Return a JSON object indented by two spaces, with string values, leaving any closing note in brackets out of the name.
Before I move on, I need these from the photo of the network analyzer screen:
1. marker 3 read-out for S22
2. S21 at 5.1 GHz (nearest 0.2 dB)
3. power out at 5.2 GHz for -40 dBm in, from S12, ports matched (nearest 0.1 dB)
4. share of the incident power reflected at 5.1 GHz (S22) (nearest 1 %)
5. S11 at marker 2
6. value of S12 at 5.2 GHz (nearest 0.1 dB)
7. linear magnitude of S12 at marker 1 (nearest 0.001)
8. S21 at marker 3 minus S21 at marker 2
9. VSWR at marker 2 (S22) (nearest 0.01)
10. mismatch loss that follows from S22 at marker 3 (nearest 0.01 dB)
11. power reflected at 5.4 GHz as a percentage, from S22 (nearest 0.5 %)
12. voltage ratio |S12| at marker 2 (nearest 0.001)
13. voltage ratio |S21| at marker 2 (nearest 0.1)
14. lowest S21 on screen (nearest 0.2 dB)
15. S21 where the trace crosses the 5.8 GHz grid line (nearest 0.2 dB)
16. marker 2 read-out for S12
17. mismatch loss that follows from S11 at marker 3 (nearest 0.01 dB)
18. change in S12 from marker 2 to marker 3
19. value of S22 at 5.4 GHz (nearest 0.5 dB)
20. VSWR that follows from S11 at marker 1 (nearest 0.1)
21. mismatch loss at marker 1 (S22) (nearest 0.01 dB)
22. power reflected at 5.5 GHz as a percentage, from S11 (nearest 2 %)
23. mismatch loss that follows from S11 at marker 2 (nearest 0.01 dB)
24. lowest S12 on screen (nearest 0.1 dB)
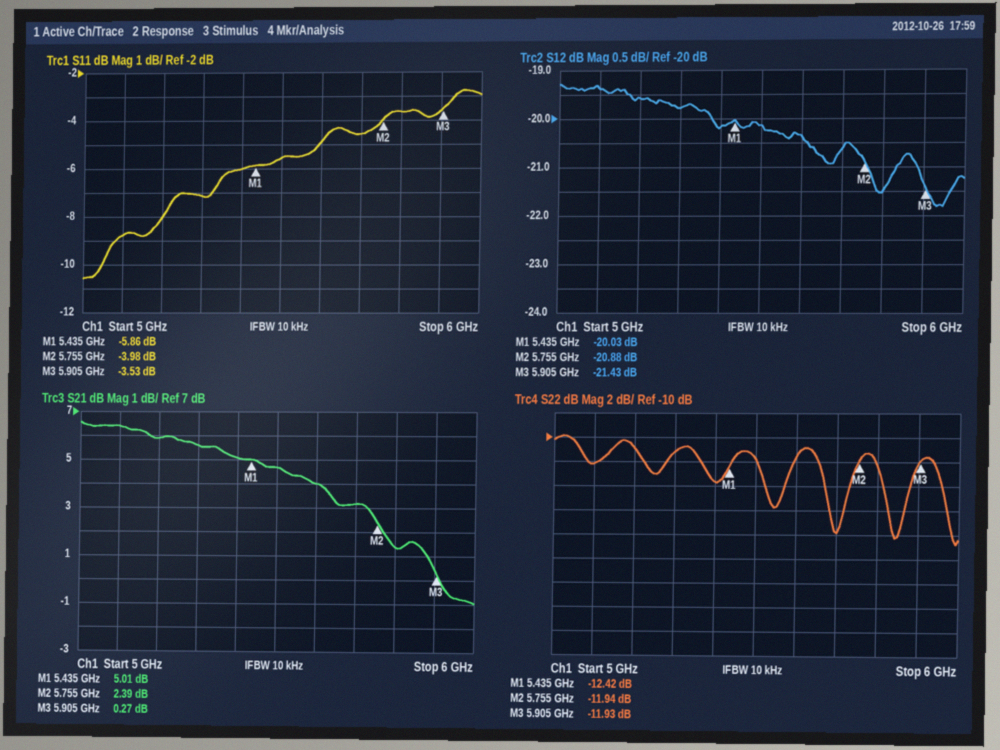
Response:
{
  "marker 3 read-out for S22": "-11.93 dB",
  "S21 at 5.1 GHz": "6.4 dB",
  "power out at 5.2 GHz for -40 dBm in, from S12, ports matched": "-59.6 dBm",
  "share of the incident power reflected at 5.1 GHz (S22)": "6 %",
  "S11 at marker 2": "-3.98 dB",
  "value of S12 at 5.2 GHz": "-19.6 dB",
  "linear magnitude of S12 at marker 1": "0.100",
  "S21 at marker 3 minus S21 at marker 2": "-2.12 dB",
  "VSWR at marker 2 (S22)": "1.68",
  "mismatch loss that follows from S22 at marker 3": "0.29 dB",
  "power reflected at 5.4 GHz as a percentage, from S22": "4.5 %",
  "voltage ratio |S12| at marker 2": "0.090",
  "voltage ratio |S21| at marker 2": "1.3",
  "lowest S21 on screen": "-1.0 dB",
  "S21 where the trace crosses the 5.8 GHz grid line": "1.4 dB",
  "marker 2 read-out for S12": "-20.88 dB",
  "mismatch loss that follows from S11 at marker 3": "2.55 dB",
  "change in S12 from marker 2 to marker 3": "-0.55 dB",
  "value of S22 at 5.4 GHz": "-13.5 dB",
  "VSWR that follows from S11 at marker 1": "3.1",
  "mismatch loss at marker 1 (S22)": "0.26 dB",
  "power reflected at 5.5 GHz as a percentage, from S11": "28 %",
  "mismatch loss that follows from S11 at marker 2": "2.22 dB",
  "lowest S12 on screen": "-21.8 dB"
}
